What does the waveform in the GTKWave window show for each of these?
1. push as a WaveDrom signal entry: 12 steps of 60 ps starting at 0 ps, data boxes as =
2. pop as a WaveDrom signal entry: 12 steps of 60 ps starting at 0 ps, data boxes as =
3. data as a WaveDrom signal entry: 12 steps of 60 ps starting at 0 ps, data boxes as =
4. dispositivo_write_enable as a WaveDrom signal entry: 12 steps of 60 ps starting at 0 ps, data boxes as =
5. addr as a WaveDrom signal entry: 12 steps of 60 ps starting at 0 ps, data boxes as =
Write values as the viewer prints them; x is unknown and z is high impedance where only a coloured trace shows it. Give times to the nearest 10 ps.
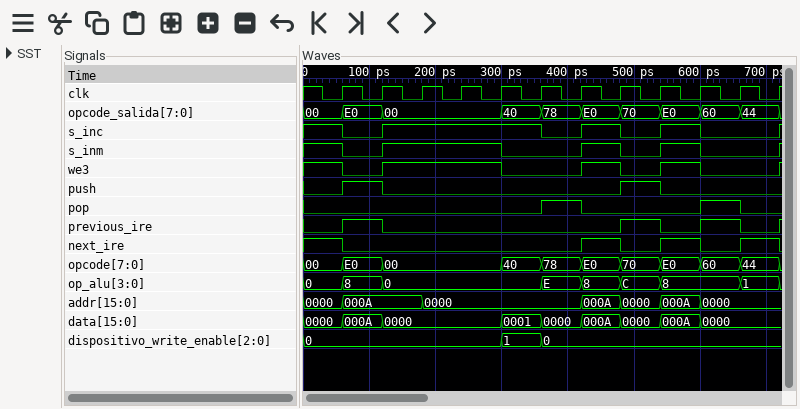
{name: 'push', wave: '010.....10..'}
{name: 'pop', wave: '0.....10..10'}
{name: 'data', wave: '===..======.', data: '0000 000A 0000 0001 0000 000A 0000 000A 0000'}
{name: 'dispositivo_write_enable', wave: '=....==.....', data: '0 1 0'}
{name: 'addr', wave: '==.=...====.', data: '0000 000A 0000 000A 0000 000A 0000'}
